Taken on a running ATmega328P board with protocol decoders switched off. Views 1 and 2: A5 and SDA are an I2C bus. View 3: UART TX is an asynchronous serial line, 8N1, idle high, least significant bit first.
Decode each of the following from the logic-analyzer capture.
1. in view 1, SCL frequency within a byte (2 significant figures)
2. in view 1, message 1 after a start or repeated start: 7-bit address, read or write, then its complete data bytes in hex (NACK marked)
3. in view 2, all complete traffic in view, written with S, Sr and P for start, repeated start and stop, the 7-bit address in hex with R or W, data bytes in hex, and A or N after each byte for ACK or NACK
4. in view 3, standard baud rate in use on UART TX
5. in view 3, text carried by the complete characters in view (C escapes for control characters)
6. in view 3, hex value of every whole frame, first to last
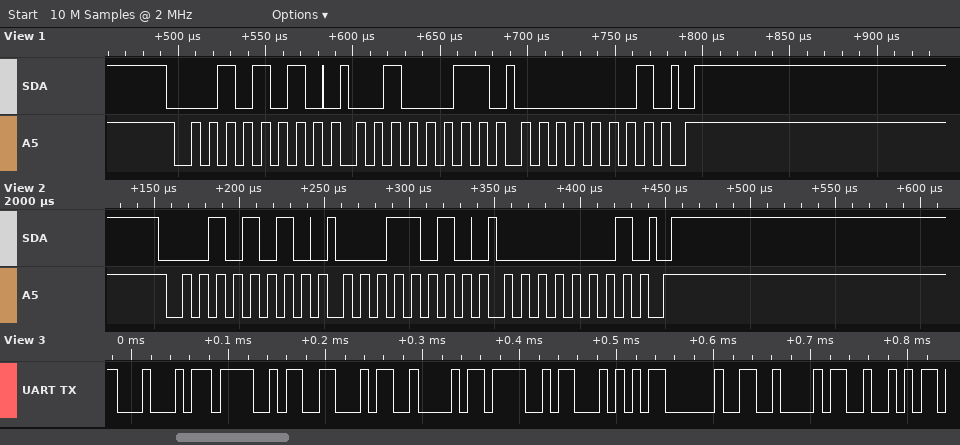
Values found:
100 kHz
0x15 write: 23 01
S 15W A 1A A 01 A P
115200 baud
"DOFBOT BR"
44 4F 46 42 4F 54 20 42 52
